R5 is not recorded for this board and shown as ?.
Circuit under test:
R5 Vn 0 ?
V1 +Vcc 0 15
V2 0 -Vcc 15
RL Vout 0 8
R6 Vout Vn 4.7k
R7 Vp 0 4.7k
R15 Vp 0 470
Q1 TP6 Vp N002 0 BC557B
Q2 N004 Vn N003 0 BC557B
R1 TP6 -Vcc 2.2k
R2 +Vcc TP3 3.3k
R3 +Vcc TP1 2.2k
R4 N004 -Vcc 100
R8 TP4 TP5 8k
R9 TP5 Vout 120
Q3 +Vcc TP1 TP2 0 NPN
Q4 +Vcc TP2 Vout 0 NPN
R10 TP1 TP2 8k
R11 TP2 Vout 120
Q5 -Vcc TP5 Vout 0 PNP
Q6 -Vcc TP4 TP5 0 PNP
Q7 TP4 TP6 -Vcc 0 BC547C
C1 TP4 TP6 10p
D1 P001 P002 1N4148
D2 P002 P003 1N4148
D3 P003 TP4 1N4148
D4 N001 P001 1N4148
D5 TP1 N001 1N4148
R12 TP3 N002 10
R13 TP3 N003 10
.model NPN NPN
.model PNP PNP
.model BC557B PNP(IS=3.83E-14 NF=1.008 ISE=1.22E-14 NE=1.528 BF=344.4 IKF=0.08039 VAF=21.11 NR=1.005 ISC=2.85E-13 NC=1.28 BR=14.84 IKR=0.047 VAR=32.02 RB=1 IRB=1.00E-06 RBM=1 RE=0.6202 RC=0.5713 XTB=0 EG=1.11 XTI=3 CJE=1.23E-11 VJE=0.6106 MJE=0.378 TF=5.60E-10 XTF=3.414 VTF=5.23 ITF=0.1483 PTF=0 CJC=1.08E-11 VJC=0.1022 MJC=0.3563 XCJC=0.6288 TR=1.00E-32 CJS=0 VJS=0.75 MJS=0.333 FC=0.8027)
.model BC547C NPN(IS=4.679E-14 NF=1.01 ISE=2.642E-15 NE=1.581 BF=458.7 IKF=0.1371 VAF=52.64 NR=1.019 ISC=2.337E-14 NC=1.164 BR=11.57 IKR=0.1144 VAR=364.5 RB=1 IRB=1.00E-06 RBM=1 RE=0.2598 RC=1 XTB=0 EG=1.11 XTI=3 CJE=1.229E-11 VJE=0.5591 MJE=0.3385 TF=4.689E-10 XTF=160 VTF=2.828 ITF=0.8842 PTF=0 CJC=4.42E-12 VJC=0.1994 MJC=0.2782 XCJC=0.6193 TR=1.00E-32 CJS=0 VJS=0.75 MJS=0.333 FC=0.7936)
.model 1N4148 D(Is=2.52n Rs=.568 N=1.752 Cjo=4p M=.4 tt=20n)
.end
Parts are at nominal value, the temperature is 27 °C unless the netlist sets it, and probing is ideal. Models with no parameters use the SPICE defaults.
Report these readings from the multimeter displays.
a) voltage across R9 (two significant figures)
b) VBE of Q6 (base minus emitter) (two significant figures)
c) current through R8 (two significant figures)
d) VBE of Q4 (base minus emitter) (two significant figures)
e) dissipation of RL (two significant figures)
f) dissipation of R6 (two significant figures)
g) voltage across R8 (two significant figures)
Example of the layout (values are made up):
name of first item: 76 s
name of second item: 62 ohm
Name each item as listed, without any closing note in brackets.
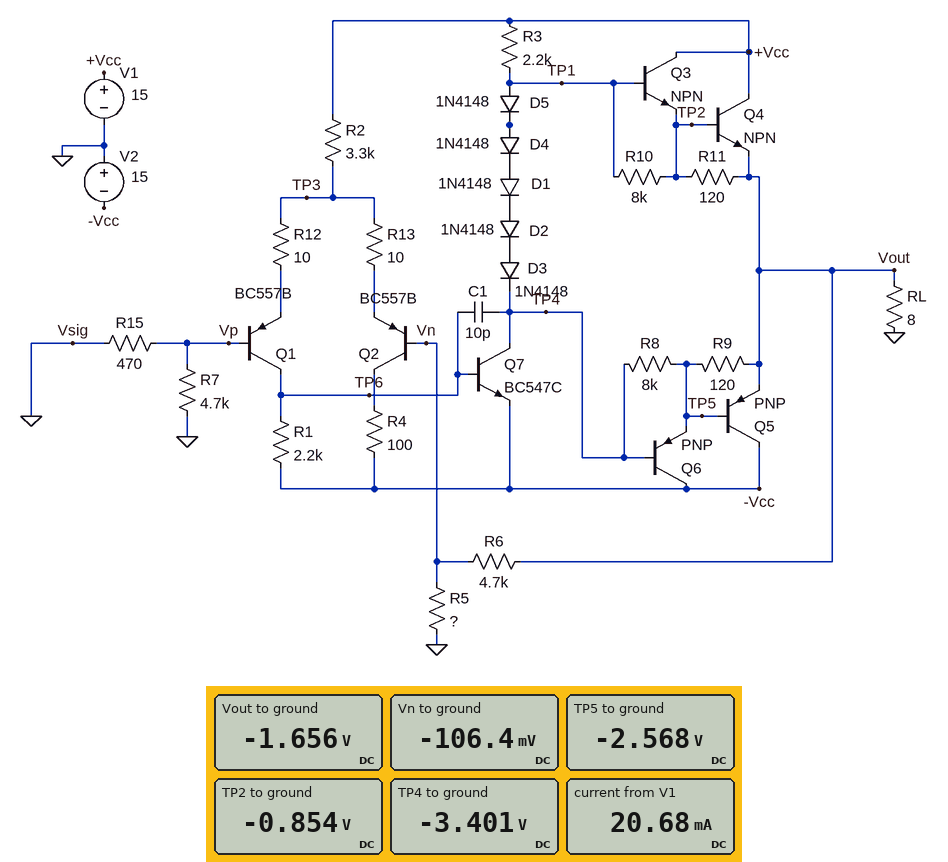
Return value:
voltage across R9: 910 mV
VBE of Q6 (base minus emitter): -830 mV
current through R8: 100 µA
VBE of Q4 (base minus emitter): 800 mV
dissipation of RL: 340 mW
dissipation of R6: 510 µW
voltage across R8: 830 mV
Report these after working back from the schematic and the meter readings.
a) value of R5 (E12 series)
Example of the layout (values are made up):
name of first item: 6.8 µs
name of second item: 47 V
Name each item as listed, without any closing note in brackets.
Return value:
value of R5: 330 Ω
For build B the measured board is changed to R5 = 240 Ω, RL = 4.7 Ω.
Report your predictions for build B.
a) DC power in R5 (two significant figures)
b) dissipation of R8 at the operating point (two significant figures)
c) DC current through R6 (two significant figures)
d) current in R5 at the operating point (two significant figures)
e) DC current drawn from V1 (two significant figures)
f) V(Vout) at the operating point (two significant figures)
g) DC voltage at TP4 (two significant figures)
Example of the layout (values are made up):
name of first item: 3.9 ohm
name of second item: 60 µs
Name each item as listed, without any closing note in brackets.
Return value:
DC power in R5: 47 µW
dissipation of R8 at the operating point: 88 µW
DC current through R6: 450 µA
current in R5 at the operating point: 440 µA
DC current drawn from V1: 19 mA
V(Vout) at the operating point: -2.2 V
DC voltage at TP4: -4.0 V
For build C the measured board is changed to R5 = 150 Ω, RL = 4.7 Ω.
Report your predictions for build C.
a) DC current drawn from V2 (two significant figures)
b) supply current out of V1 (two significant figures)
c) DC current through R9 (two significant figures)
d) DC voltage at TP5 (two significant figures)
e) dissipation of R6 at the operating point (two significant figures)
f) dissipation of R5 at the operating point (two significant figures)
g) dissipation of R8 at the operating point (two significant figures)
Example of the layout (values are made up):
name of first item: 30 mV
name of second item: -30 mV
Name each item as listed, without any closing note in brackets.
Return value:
DC current drawn from V2: 760 mA
supply current out of V1: 20 mA
DC current through R9: 7.9 mA
DC voltage at TP5: -4.4 V
dissipation of R6 at the operating point: 2.4 mW
dissipation of R5 at the operating point: 75 µW
dissipation of R8 at the operating point: 89 µW
